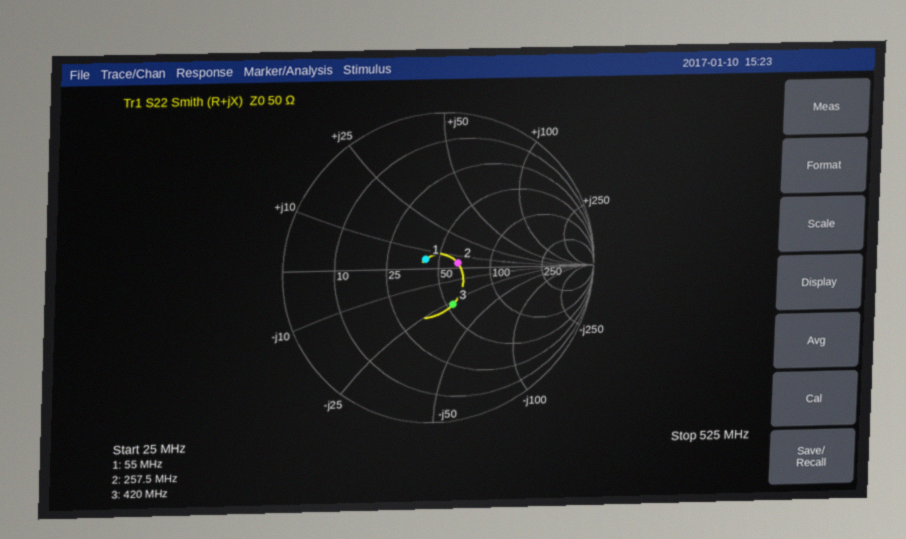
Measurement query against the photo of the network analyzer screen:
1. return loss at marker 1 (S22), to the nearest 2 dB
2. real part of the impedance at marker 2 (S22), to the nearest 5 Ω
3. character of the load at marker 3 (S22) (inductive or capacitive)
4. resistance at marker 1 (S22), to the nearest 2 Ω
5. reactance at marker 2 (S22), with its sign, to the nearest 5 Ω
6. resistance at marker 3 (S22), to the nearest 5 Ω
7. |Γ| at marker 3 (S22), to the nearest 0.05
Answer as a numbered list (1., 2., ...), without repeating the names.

1. 20 dB
2. 65 Ω
3. capacitive
4. 42 Ω
5. +5 Ω
6. 55 Ω
7. 0.25
